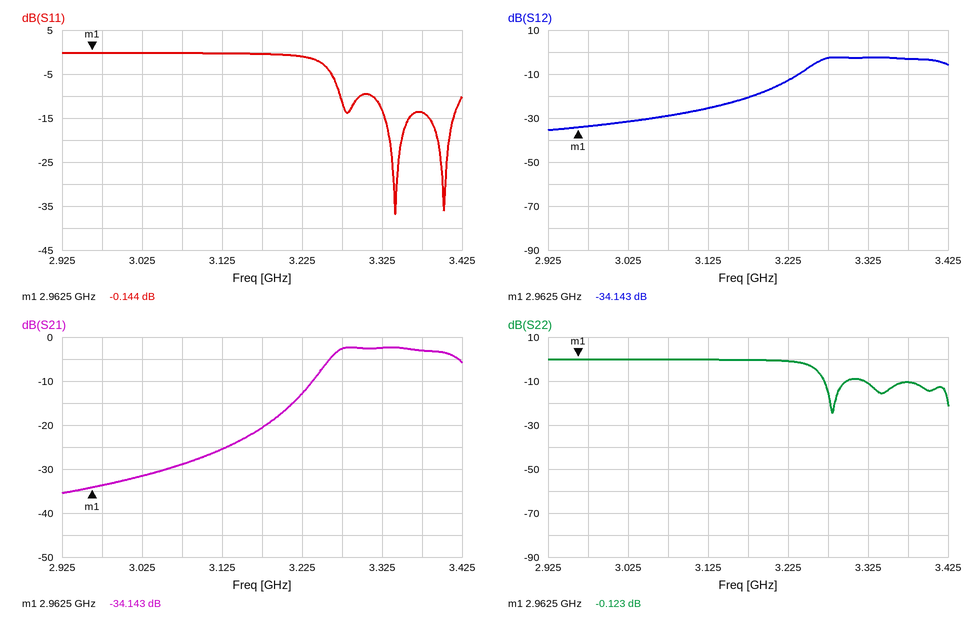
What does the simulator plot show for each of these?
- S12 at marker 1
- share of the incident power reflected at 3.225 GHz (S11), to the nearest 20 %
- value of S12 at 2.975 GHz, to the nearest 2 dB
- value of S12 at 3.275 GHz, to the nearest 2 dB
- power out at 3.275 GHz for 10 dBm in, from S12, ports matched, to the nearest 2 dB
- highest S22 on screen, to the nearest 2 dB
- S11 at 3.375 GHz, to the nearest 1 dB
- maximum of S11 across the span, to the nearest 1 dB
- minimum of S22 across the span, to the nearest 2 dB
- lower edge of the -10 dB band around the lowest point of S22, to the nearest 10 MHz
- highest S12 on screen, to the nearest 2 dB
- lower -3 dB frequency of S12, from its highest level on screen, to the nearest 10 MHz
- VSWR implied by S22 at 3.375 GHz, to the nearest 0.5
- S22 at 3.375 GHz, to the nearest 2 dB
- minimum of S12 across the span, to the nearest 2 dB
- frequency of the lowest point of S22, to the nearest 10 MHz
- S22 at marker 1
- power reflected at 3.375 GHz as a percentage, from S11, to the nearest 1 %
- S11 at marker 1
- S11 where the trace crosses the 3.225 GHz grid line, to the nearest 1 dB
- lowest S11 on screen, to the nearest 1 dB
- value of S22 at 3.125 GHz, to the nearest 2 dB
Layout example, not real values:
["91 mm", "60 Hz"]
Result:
["-34.143 dB", "80 %", "-34 dB", "-2 dB", "8 dBm", "0 dB", "-14 dB", "0 dB", "-24 dB", "3.27 GHz", "-2 dB", "3.26 GHz", "2.0", "-10 dB", "-36 dB", "3.28 GHz", "-0.123 dB", "4 %", "-0.144 dB", "-1 dB", "-37 dB", "0 dB"]
